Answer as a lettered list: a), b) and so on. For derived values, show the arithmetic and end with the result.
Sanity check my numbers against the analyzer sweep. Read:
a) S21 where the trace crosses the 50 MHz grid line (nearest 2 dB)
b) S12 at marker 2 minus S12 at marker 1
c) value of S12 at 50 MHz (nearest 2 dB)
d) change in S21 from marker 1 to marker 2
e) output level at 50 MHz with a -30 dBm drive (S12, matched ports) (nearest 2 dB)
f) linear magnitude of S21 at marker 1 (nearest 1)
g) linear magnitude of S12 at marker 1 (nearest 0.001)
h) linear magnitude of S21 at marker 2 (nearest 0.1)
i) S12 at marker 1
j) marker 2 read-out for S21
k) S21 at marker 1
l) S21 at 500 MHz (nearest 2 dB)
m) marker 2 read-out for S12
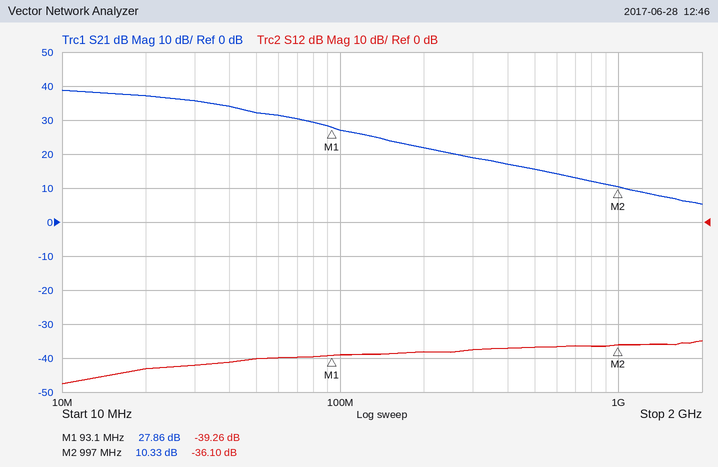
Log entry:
a) 32 dB
b) -36.1 − (-39.26) = 3.16 dB
c) -40 dB
d) 10.33 − (27.86) = -17.53 dB
e) -30 dBm + (-40 dB) = -70 dBm
f) 10^(27.86/20) ≈ 25
g) 10^(-39.26/20) ≈ 0.011
h) 10^(10.33/20) ≈ 3.3
i) -39.26 dB
j) 10.33 dB
k) 27.86 dB
l) 16 dB
m) -36.10 dB
